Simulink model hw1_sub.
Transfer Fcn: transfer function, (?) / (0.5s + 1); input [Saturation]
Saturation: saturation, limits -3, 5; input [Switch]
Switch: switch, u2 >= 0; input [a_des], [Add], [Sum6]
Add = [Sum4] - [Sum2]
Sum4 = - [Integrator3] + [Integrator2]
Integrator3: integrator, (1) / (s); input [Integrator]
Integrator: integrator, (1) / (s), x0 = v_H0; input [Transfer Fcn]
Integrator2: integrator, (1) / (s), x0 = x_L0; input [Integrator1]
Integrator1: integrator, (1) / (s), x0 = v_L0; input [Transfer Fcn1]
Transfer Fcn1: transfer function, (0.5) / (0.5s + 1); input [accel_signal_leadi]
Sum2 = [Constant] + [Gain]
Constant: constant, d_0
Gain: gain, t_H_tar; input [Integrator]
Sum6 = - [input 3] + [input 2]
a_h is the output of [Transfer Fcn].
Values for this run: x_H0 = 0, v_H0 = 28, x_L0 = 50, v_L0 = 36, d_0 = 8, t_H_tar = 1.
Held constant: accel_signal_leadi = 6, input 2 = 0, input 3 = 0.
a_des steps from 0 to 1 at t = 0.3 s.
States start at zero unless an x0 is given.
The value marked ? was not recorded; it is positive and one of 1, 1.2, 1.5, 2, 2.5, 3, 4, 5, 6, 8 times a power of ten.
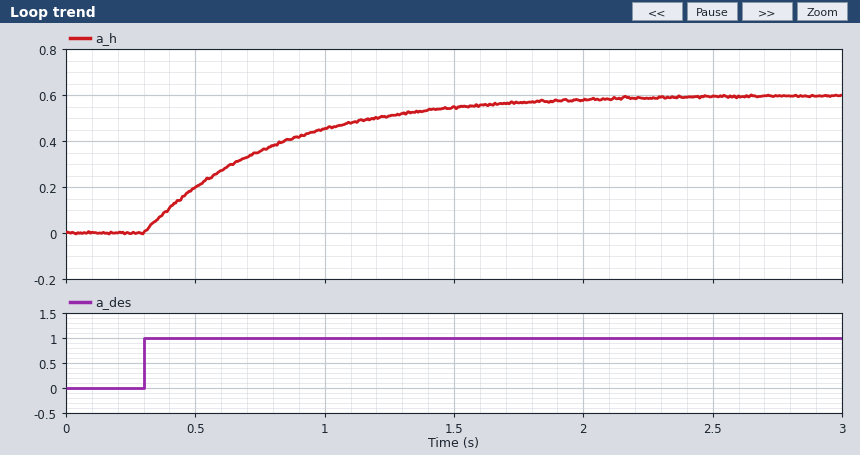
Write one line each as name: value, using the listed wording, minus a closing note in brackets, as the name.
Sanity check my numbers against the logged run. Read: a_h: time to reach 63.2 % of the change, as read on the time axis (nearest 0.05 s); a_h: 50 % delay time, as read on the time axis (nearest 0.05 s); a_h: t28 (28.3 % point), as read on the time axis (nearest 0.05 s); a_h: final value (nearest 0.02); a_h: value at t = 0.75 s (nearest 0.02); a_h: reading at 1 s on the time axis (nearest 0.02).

a_h: time to reach 63.2 % of the change, as read on the time axis: 0.80 s
a_h: 50 % delay time, as read on the time axis: 0.65 s
a_h: t28 (28.3 % point), as read on the time axis: 0.45 s
a_h: final value: 0.60
a_h: value at t = 0.75 s: 0.36
a_h: reading at 1 s on the time axis: 0.46
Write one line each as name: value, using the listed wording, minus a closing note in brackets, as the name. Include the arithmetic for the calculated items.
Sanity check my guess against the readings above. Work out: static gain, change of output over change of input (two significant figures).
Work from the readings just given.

static gain, change of output over change of input: (0.6 - 0) / (1 - 0) = 0.60
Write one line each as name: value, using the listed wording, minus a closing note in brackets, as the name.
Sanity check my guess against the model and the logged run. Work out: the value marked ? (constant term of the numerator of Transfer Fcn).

the value marked ?: 0.6
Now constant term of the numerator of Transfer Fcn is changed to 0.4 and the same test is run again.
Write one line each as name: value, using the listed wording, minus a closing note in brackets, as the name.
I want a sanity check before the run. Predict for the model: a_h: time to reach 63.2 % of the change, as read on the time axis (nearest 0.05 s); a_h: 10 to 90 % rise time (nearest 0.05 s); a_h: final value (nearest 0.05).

a_h: time to reach 63.2 % of the change, as read on the time axis: 0.80 s
a_h: 10 to 90 % rise time: 1.10 s
a_h: final value: 0.40
